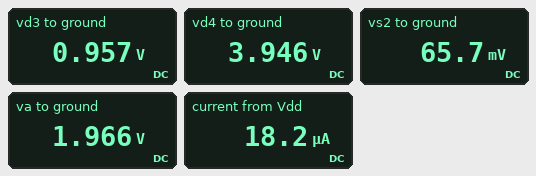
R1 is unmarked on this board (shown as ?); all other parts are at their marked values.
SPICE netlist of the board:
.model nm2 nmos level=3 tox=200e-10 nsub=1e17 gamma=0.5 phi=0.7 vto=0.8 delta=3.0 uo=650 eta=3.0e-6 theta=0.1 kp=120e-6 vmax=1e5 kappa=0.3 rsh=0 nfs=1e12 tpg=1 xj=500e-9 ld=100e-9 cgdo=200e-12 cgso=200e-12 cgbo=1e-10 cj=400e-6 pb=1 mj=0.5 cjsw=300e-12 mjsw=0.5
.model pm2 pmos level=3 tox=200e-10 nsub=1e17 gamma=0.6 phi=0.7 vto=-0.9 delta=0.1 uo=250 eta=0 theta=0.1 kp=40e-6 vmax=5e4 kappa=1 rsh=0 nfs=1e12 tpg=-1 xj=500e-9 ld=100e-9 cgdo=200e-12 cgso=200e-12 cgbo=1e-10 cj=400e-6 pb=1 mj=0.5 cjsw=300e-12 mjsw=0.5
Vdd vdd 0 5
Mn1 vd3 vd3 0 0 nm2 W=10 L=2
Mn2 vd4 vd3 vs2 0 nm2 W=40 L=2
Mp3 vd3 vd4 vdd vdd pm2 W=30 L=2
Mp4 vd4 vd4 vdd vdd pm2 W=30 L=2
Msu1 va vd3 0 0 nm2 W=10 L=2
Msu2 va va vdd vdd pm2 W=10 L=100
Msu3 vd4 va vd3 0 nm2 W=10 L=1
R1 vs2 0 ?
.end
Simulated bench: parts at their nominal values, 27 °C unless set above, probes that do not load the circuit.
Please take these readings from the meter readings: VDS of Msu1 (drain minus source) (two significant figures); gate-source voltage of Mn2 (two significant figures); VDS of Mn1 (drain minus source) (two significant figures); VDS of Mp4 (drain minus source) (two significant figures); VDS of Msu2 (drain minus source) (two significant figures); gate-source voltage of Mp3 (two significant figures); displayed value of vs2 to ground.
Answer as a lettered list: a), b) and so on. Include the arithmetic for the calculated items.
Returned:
a) 1.966 V = 2.0 V
b) 957 mV - 65.7 mV = 890 mV
c) 957 mV = 960 mV
d) 3.946 V - 5 V = -1.1 V
e) 1.966 V - 5 V = -3.0 V
f) 3.946 V - 5 V = -1.1 V
g) 65.7 mV
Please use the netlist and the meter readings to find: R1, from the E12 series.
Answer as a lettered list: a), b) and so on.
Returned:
a) 12 kΩ
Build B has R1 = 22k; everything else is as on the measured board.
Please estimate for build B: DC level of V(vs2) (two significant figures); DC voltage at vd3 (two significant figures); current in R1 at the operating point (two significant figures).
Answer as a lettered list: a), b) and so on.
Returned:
a) 75 mV
b) 950 mV
c) 3.4 µA
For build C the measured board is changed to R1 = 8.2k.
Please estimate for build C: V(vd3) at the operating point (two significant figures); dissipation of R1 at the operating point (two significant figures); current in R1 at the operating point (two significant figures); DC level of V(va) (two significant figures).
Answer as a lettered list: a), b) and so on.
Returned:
a) 990 mV
b) 640 nW
c) 8.8 µA
d) 1.5 V
